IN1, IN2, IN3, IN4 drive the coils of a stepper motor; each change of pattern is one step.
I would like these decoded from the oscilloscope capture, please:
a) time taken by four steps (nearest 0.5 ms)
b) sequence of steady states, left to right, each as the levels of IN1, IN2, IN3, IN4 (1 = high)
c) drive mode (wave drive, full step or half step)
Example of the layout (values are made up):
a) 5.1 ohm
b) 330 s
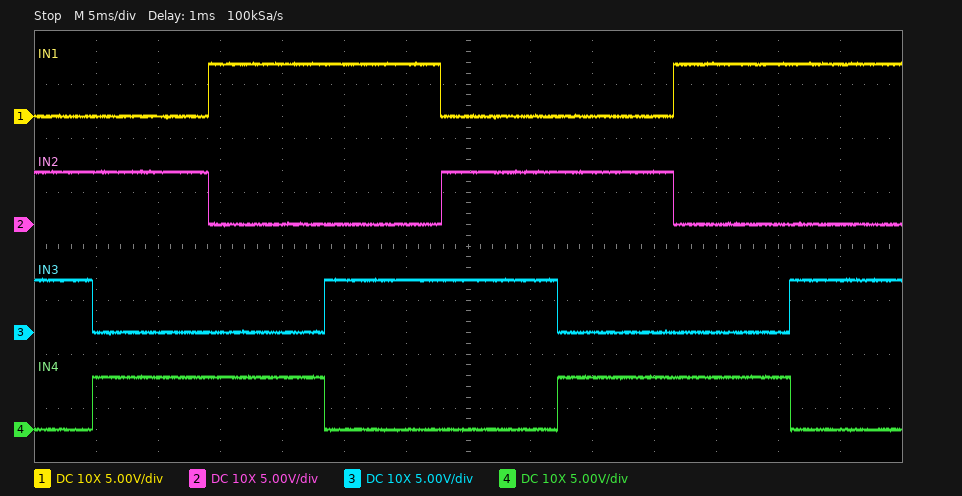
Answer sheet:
a) 37.5 ms
b) 0110 0101 1001 1010 0110 0101 1001 1010
c) full step
